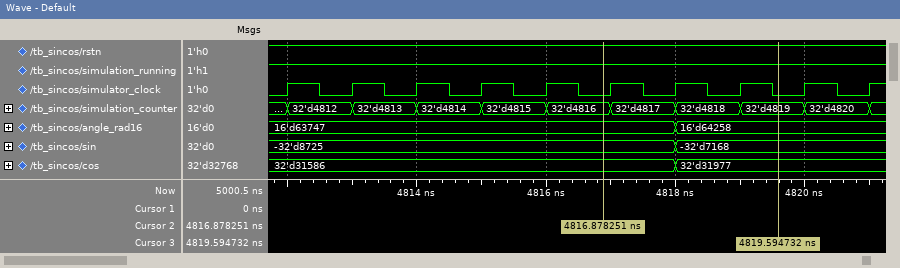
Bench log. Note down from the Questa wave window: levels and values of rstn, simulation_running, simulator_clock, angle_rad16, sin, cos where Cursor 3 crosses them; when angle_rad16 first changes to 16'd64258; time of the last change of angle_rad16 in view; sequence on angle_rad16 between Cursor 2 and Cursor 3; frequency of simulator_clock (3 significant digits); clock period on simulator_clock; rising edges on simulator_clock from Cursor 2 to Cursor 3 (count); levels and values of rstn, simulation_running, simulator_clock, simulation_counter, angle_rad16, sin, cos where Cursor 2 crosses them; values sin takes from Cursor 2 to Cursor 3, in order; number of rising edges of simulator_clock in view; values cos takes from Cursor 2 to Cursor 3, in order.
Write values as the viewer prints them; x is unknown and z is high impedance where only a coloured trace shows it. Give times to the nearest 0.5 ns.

rstn=1, simulation_running=1, simulator_clock=0, angle_rad16=16'd64258, sin=-32'd7168, cos=32'd31977
4818 ns
4818 ns
16'd63747, 16'd64258
1.00 GHz
1 ns
3
rstn=1, simulation_running=1, simulator_clock=0, simulation_counter=32'd4816, angle_rad16=16'd63747, sin=-32'd8725, cos=32'd31586
-32'd8725, -32'd7168
10
32'd31586, 32'd31977
